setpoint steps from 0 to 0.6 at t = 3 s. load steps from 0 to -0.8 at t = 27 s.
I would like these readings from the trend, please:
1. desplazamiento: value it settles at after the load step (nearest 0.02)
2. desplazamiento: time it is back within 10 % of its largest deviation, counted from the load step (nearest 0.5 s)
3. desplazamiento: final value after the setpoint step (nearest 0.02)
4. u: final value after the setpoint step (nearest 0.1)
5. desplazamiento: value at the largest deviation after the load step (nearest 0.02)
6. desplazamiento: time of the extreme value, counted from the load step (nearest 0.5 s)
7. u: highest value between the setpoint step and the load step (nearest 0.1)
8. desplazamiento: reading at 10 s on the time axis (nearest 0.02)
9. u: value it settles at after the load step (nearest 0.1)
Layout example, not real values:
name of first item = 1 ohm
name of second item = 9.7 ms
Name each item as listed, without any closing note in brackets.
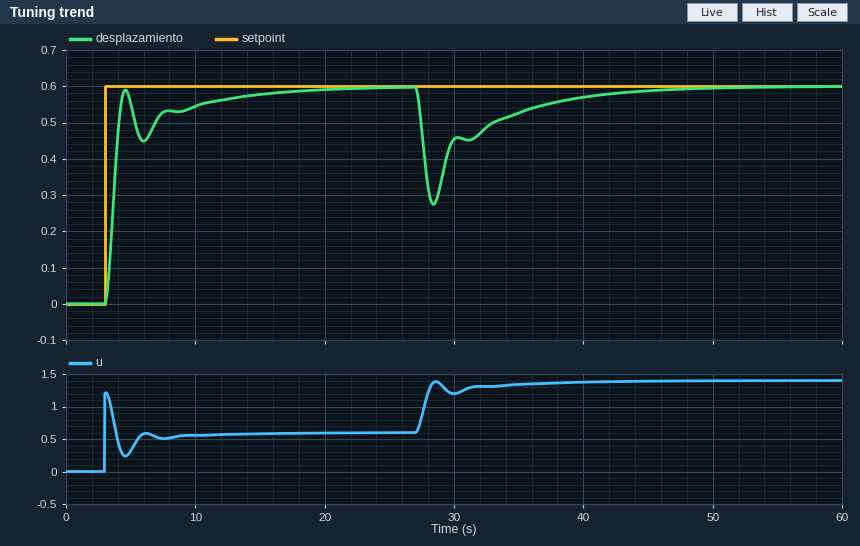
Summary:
desplazamiento: value it settles at after the load step = 0.60
desplazamiento: time it is back within 10 % of its largest deviation, counted from the load step = 12.5 s
desplazamiento: final value after the setpoint step = 0.60
u: final value after the setpoint step = 0.6
desplazamiento: value at the largest deviation after the load step = 0.28
desplazamiento: time of the extreme value, counted from the load step = 1.5 s
u: highest value between the setpoint step and the load step = 1.2
desplazamiento: reading at 10 s on the time axis = 0.54
u: value it settles at after the load step = 1.4
